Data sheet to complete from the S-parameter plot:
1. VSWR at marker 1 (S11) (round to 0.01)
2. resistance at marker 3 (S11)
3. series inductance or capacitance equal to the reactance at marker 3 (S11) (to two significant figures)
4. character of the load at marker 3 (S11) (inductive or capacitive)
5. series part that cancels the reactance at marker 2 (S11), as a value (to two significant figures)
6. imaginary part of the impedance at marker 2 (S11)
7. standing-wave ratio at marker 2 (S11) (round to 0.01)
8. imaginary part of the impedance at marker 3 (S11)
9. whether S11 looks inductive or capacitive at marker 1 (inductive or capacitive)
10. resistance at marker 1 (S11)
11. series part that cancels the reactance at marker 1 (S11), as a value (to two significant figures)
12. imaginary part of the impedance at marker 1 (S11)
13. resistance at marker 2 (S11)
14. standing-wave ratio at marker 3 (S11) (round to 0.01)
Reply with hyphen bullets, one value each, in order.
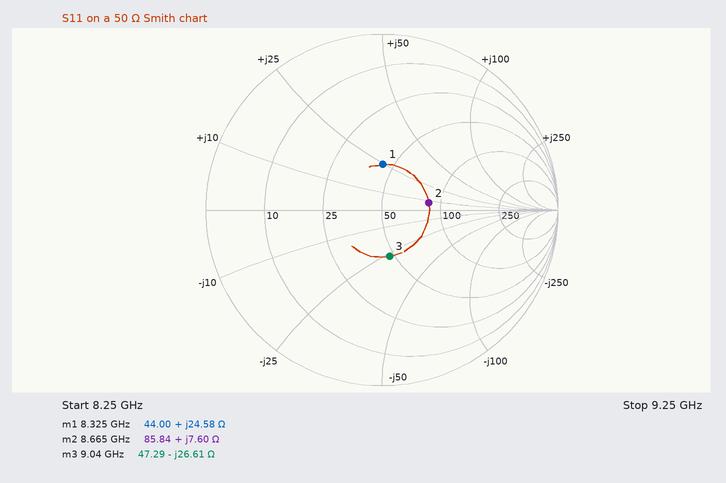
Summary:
- 1.70
- 47.29 Ω
- 660 fF
- capacitive
- 2.4 pF
- +7.60 Ω
- 1.74
- -26.61 Ω
- inductive
- 44.00 Ω
- 780 fF
- +24.58 Ω
- 85.84 Ω
- 1.72
